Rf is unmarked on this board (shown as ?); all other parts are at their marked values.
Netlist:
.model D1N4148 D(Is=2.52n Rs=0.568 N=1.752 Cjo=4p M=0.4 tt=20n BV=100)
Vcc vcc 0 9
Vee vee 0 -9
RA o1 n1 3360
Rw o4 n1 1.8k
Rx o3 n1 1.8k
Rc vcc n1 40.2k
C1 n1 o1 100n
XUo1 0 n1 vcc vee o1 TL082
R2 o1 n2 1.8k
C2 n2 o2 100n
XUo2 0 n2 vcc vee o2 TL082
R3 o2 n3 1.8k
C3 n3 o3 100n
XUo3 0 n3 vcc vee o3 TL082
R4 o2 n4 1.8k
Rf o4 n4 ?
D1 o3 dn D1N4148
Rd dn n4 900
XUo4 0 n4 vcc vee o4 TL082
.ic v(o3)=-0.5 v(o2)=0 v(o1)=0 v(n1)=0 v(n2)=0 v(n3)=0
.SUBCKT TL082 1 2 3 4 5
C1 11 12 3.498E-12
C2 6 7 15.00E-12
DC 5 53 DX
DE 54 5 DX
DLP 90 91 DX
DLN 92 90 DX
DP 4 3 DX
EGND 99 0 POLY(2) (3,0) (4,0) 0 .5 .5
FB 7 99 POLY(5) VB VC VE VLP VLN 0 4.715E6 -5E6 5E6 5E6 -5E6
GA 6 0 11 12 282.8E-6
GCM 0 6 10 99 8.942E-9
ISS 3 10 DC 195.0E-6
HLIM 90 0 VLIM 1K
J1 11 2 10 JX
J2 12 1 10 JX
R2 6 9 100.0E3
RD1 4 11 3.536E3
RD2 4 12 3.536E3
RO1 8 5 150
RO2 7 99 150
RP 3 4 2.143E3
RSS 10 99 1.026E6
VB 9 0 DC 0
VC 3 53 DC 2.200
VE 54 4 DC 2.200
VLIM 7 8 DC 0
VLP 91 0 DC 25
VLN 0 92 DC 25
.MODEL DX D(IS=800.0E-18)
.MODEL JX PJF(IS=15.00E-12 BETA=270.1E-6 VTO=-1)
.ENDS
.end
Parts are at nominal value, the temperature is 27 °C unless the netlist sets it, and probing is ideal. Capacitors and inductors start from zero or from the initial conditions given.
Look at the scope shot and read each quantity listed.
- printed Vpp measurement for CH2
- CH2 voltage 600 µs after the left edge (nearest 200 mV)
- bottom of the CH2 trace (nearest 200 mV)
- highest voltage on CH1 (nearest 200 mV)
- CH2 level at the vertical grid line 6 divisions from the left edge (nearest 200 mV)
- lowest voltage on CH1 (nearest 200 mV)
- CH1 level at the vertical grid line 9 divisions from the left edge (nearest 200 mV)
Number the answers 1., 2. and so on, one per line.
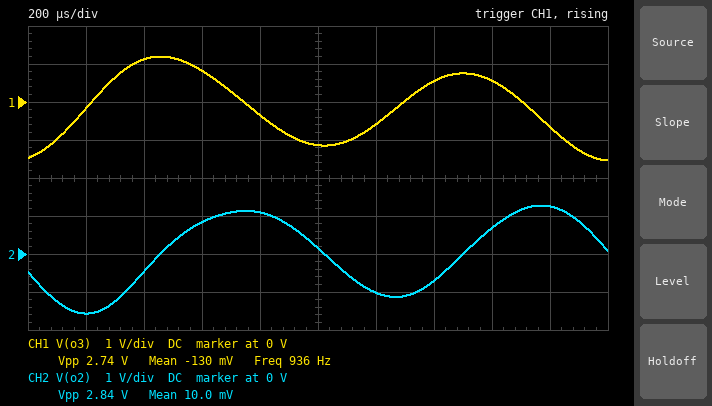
1. 2.84 V
2. 800 mV
3. -1.6 V
4. 1.2 V
5. -1.0 V
6. -1.6 V
7. -600 mV
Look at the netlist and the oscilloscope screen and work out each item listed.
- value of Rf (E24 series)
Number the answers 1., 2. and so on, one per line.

1. 2.2 kΩ
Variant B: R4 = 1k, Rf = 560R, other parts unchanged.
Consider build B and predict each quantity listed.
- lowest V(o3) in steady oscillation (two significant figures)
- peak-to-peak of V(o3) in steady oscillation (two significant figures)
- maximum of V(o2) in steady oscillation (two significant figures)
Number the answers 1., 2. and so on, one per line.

1. -7.5 V
2. 15 V
3. 7.5 V
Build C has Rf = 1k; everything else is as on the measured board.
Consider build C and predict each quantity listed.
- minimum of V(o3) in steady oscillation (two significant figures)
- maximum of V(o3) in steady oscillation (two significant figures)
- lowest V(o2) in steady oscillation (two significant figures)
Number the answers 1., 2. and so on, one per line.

1. -3.1 V
2. 7.4 V
3. -4.3 V
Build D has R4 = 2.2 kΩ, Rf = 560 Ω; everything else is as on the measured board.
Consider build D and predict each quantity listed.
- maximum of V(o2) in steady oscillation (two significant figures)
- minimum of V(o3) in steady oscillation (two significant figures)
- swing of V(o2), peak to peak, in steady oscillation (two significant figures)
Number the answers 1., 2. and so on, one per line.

1. 7.5 V
2. -7.5 V
3. 15 V
